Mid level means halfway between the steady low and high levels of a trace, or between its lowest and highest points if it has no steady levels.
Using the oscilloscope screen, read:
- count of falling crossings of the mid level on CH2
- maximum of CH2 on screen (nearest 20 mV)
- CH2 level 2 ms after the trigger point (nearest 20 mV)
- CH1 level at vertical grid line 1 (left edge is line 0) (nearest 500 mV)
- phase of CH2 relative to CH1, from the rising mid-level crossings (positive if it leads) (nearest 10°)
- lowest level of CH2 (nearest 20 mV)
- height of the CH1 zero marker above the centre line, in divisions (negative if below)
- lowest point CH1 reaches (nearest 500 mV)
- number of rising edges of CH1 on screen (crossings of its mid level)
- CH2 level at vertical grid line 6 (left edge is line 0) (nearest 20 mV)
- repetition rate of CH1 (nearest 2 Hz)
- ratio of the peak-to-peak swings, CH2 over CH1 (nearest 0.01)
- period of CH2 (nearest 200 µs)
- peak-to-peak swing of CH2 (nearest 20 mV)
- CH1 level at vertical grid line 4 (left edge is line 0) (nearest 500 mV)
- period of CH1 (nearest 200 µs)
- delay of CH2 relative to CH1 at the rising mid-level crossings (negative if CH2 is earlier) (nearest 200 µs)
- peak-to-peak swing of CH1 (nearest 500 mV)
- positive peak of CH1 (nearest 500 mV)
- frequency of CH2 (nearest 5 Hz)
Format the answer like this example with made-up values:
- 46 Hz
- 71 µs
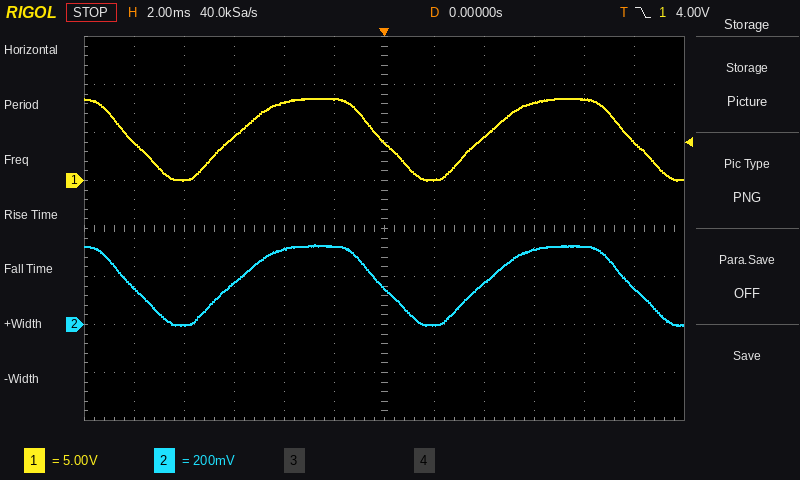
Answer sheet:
- 3
- 340 mV
- 0 mV
- 4.0 V
- 0°
- 0 mV
- +1.0 div
- 0.0 V
- 2
- 160 mV
- 100 Hz
- 0.04
- 10.0 ms
- 340 mV
- 8.0 V
- 10.0 ms
- 0.0 ms
- 8.5 V
- 8.5 V
- 100 Hz
